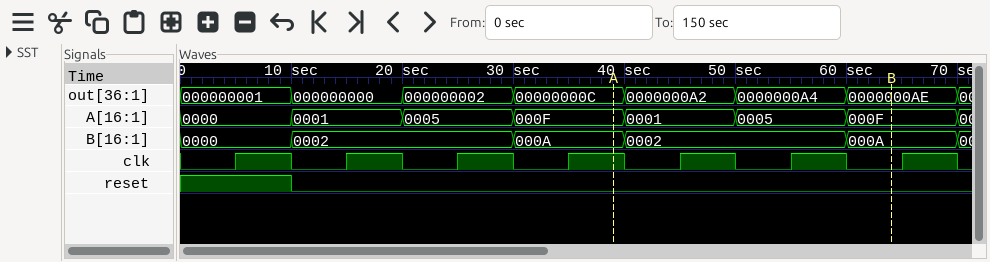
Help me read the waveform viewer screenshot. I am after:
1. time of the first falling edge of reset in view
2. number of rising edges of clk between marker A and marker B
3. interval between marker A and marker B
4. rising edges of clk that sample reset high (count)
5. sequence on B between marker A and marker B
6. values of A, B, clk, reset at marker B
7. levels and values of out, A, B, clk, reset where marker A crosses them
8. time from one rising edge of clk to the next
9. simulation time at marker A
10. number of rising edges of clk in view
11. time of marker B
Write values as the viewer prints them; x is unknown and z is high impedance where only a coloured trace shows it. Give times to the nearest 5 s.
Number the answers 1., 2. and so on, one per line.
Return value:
1. 10 s
2. 2
3. 25 s
4. 1
5. 000A, 0002, 000A
6. A=000F, B=000A, clk=0, reset=0
7. out=00000000C, A=000F, B=000A, clk=1, reset=0
8. 10 s
9. 40 s
10. 7
11. 65 s
